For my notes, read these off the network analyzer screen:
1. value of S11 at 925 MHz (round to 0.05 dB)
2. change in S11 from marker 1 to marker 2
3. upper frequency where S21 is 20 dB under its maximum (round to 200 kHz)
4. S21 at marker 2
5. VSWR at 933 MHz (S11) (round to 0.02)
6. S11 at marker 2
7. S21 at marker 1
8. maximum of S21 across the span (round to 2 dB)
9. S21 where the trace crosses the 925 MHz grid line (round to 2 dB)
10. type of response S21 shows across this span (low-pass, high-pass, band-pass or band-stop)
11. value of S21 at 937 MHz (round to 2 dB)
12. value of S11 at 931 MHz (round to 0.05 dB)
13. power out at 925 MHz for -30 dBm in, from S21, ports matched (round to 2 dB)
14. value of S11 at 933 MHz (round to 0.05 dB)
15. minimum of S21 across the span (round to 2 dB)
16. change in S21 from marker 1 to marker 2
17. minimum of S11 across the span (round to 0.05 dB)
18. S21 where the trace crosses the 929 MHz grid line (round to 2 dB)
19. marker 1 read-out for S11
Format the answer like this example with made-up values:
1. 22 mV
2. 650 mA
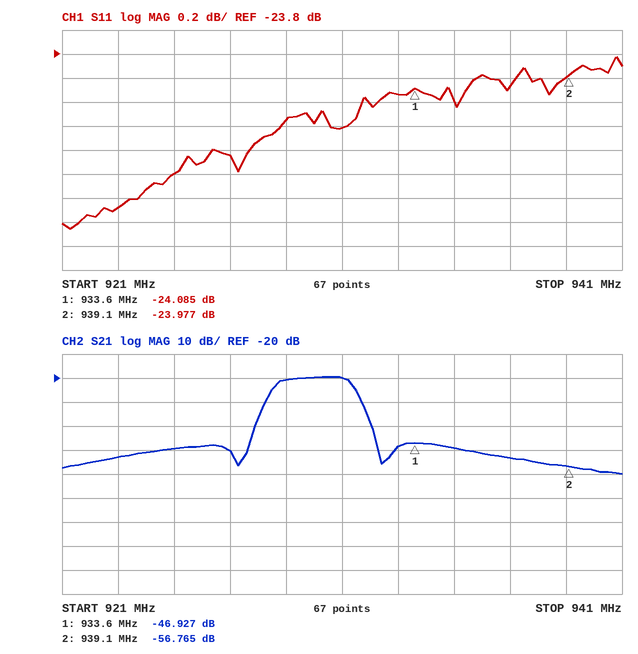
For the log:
1. -24.80 dB
2. 0.108 dB
3. 932.0 MHz
4. -56.765 dB
5. 1.14
6. -23.977 dB
7. -46.927 dB
8. -20 dB
9. -50 dB
10. band-pass
11. -54 dB
12. -24.40 dB
13. -80 dBm
14. -24.15 dB
15. -60 dB
16. -9.838 dB
17. -25.25 dB
18. -20 dB
19. -24.085 dB
